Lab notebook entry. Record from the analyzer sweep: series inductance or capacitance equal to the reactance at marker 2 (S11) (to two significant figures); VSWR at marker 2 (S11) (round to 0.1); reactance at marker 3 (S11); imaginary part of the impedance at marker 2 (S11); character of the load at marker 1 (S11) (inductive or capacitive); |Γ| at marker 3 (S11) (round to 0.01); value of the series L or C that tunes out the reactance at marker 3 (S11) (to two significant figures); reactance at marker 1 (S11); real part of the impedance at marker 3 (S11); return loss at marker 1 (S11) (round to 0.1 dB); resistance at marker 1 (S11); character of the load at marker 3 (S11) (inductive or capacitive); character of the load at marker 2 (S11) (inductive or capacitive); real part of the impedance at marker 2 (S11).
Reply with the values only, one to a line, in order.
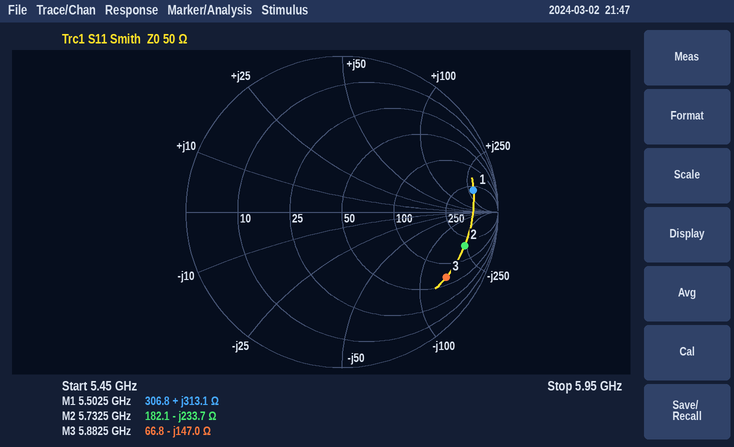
120 fF
9.8
-147.0 Ω
-233.7 Ω
inductive
0.79
4.0 nH
+313.1 Ω
66.8 Ω
1.4 dB
306.8 Ω
capacitive
capacitive
182.1 Ω
